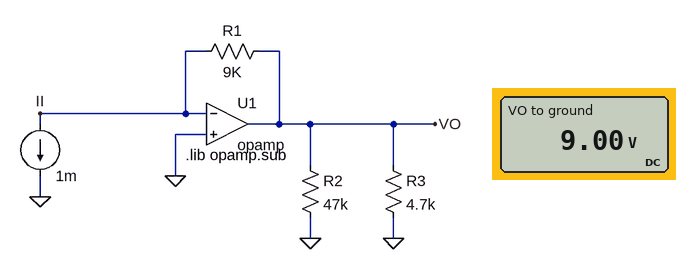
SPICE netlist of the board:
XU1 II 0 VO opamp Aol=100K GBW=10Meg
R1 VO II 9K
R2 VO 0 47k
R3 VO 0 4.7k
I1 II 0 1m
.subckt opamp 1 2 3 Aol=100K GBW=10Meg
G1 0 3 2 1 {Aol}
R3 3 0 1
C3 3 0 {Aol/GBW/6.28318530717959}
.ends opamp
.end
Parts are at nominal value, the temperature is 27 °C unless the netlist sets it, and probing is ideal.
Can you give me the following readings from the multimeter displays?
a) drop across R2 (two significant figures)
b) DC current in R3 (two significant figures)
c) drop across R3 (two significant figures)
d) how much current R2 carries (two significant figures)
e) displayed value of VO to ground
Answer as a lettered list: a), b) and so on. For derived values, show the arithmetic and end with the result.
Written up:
a) 9 V = 9.0 V
b) (9 V) / 4.7 kΩ = 1.9 mA
c) 9 V = 9.0 V
d) (9 V) / 47 kΩ = 190 µA
e) 9.00 V
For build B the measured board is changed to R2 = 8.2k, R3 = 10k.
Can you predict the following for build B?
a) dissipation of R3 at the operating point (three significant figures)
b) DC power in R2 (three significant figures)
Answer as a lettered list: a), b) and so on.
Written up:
a) 8.10 mW
b) 9.88 mW
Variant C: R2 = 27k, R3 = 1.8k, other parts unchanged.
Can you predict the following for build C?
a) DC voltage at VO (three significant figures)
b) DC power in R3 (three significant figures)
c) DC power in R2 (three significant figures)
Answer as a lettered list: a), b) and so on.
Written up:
a) 9.00 V
b) 45.0 mW
c) 3.00 mW
